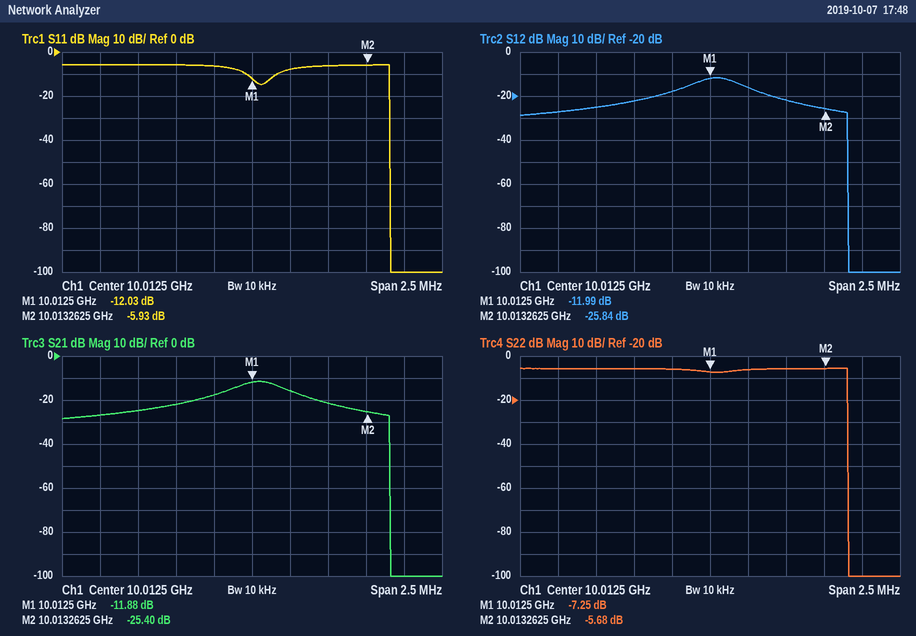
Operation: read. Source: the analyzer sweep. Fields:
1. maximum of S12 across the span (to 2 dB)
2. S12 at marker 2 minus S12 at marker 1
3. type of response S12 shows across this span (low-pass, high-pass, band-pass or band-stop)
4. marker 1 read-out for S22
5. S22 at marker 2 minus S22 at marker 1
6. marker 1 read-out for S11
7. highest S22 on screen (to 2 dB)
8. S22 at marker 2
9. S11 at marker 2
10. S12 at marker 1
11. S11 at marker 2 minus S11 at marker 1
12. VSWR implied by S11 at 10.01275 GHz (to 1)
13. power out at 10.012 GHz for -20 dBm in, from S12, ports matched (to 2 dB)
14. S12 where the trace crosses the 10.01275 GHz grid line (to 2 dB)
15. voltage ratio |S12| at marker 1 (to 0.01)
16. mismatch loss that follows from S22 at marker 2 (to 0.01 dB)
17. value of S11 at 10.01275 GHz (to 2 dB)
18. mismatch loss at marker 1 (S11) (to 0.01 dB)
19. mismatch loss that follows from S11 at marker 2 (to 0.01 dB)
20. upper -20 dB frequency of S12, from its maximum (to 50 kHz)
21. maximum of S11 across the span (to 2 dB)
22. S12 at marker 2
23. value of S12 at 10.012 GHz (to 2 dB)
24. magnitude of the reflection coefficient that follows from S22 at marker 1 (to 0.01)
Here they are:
-12 dB
-13.85 dB
band-pass
-7.25 dB
1.57 dB
-12.03 dB
-6 dB
-5.68 dB
-5.93 dB
-11.99 dB
6.10 dB
2
-42 dBm
-16 dB
0.25
1.37 dB
-8 dB
0.28 dB
1.28 dB
10.01340 GHz
-6 dB
-25.84 dB
-22 dB
0.43
